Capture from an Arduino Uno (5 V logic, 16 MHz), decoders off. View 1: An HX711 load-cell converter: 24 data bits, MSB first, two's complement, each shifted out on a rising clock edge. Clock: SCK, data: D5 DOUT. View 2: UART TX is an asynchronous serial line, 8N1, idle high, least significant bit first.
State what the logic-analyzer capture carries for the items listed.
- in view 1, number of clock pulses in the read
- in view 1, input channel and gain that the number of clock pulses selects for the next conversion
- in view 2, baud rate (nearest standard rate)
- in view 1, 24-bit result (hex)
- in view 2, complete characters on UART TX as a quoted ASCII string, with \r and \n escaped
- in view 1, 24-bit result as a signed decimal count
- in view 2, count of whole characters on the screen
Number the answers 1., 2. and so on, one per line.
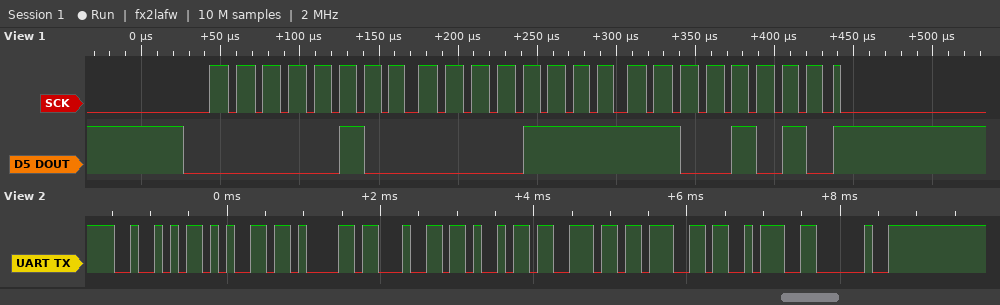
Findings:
1. 25
2. channel A, gain 128
3. 9600 baud
4. 0x040FCA
5. "Reading: "
6. 266186
7. 9
